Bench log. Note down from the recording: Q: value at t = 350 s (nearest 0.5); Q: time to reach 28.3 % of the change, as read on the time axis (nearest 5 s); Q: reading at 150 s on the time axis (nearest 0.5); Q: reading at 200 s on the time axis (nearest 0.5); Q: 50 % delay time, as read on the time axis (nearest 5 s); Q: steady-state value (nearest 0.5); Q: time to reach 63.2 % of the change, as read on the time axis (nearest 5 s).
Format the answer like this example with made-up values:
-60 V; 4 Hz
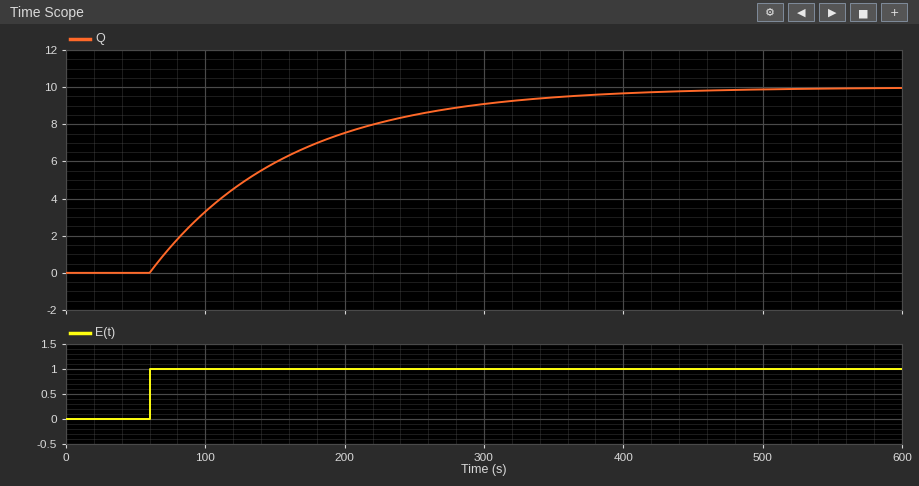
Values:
9.5; 95 s; 6.0; 7.5; 130 s; 10.0; 160 s
